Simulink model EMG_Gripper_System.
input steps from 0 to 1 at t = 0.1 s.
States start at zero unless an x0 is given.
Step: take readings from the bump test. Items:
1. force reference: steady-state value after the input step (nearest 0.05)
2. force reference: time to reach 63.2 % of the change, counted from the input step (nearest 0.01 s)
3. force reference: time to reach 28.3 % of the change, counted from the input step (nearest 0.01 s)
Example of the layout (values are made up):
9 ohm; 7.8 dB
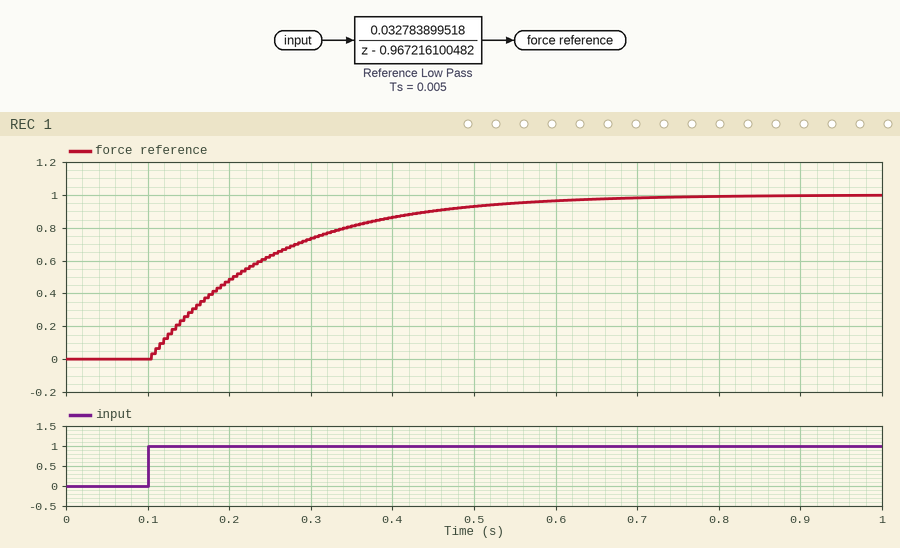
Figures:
1.00; 0.15 s; 0.05 s
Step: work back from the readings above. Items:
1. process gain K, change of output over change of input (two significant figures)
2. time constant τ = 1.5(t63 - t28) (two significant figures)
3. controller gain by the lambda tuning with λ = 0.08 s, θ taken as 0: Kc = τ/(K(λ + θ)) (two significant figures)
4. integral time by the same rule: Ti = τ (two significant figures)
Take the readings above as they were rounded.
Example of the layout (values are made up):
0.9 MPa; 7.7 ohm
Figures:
1.0; 0.15 s; 1.9; 0.15 s
